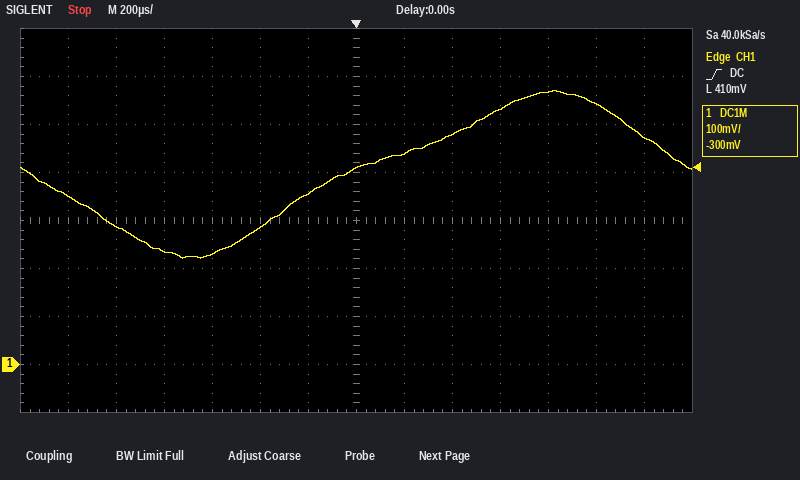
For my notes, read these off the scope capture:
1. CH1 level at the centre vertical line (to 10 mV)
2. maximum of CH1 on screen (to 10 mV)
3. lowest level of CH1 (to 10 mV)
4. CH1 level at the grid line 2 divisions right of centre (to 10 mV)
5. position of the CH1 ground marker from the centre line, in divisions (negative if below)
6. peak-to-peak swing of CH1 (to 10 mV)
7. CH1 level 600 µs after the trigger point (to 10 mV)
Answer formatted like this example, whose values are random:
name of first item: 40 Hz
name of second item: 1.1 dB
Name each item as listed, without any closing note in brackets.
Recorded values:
CH1 level at the centre vertical line: 410 mV
maximum of CH1 on screen: 570 mV
lowest level of CH1: 220 mV
CH1 level at the grid line 2 divisions right of centre: 480 mV
position of the CH1 ground marker from the centre line, in divisions: -3.0 div
peak-to-peak swing of CH1: 350 mV
CH1 level 600 µs after the trigger point: 530 mV
